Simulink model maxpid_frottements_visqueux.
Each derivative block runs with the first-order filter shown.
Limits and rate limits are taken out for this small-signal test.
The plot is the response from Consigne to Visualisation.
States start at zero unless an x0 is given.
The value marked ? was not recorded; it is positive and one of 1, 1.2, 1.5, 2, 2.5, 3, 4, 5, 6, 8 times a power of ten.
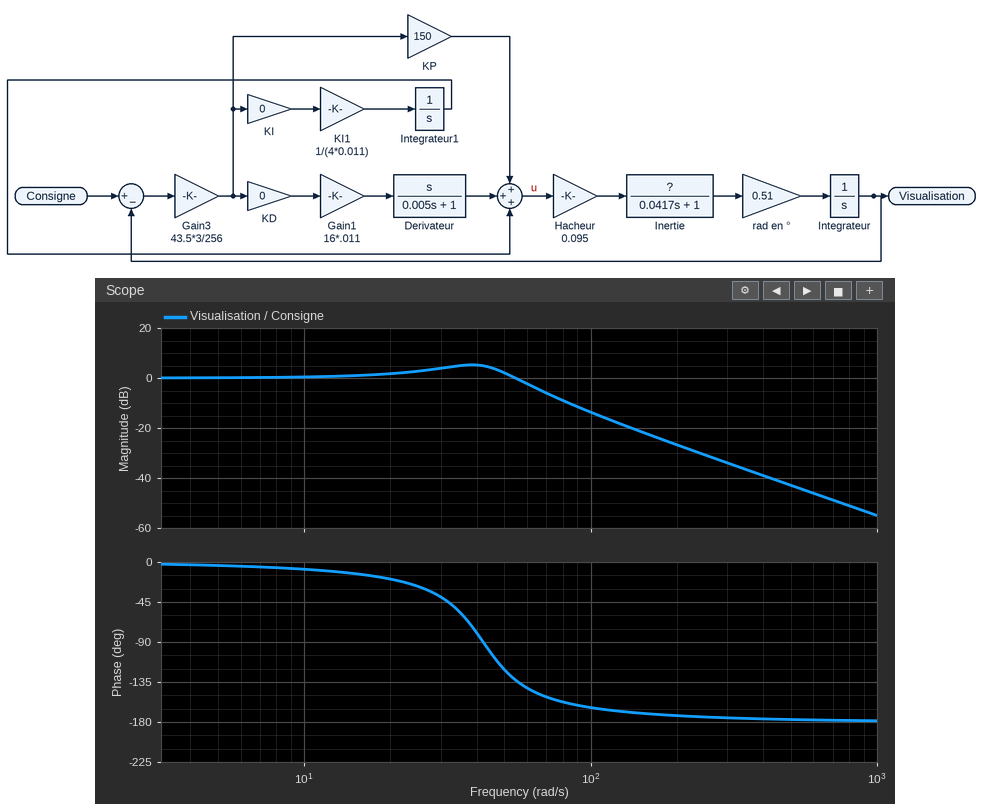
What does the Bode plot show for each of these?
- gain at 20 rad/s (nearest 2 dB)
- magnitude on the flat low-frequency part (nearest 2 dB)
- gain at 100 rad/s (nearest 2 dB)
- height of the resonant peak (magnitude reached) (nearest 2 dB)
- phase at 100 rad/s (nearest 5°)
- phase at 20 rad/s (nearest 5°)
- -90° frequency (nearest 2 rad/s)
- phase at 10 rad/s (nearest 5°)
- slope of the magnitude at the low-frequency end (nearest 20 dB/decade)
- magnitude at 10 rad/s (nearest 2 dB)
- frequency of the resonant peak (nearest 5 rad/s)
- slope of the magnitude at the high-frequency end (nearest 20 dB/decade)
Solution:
2 dB
0 dB
-14 dB
6 dB
-165°
-20°
42 rad/s
-10°
0 dB/decade
0 dB
40 rad/s
-40 dB/decade
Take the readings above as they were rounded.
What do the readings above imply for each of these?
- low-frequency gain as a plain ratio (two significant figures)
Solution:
1.0
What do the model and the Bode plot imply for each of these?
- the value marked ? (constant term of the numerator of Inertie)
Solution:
20
